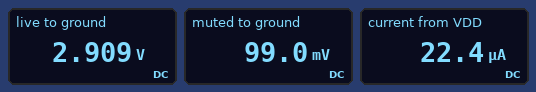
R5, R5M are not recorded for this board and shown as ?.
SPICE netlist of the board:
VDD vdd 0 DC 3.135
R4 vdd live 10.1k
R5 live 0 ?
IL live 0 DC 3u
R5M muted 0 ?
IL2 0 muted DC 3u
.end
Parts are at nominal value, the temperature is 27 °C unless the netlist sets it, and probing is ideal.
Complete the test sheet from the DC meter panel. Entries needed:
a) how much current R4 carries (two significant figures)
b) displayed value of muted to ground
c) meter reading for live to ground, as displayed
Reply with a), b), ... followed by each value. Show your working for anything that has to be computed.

a) (3.135 V - 2.909 V) / 10.1 kΩ = 22 µA
b) 99.0 mV
c) 2.909 V
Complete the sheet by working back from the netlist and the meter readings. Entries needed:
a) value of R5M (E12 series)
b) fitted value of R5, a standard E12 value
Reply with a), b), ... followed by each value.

a) 33 kΩ
b) 150 kΩ
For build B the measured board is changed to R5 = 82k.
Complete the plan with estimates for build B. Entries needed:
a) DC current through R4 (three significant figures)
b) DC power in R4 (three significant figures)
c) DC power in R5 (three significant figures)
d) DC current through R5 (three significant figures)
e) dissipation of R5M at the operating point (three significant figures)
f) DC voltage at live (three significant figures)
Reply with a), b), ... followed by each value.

a) 36.7 µA
b) 13.6 µW
c) 93.2 µW
d) 33.7 µA
e) 297 nW
f) 2.76 V
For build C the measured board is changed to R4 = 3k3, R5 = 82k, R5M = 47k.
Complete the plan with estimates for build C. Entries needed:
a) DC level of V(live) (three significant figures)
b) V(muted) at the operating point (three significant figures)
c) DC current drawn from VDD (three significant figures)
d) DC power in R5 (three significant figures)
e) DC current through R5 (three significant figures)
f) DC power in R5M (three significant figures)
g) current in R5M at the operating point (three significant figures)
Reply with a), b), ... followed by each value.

a) 3.00 V
b) 141 mV
c) 39.6 µA
d) 110 µW
e) 36.6 µA
f) 423 nW
g) 3.00 µA
